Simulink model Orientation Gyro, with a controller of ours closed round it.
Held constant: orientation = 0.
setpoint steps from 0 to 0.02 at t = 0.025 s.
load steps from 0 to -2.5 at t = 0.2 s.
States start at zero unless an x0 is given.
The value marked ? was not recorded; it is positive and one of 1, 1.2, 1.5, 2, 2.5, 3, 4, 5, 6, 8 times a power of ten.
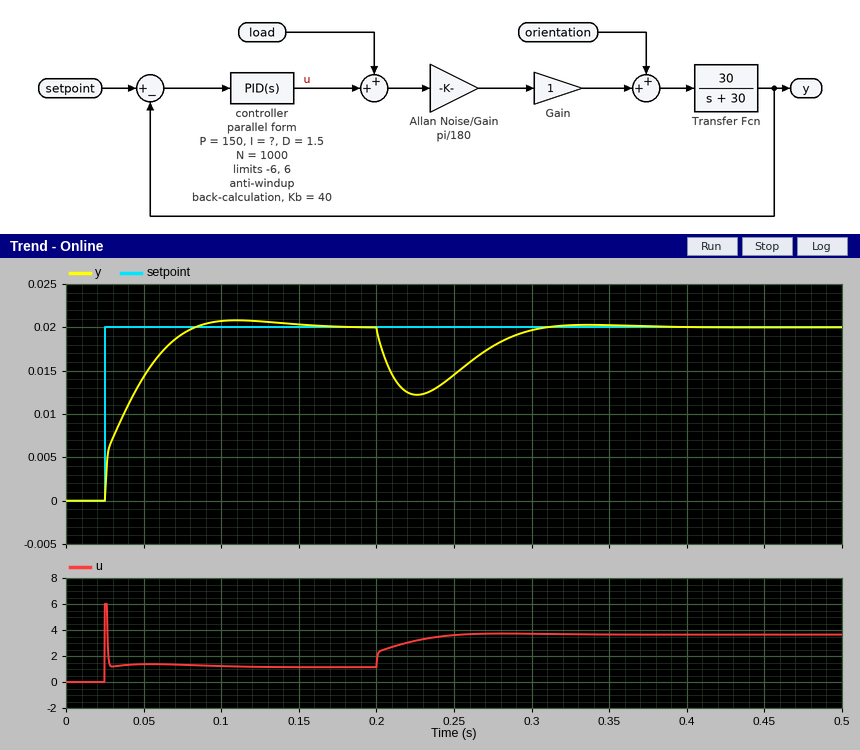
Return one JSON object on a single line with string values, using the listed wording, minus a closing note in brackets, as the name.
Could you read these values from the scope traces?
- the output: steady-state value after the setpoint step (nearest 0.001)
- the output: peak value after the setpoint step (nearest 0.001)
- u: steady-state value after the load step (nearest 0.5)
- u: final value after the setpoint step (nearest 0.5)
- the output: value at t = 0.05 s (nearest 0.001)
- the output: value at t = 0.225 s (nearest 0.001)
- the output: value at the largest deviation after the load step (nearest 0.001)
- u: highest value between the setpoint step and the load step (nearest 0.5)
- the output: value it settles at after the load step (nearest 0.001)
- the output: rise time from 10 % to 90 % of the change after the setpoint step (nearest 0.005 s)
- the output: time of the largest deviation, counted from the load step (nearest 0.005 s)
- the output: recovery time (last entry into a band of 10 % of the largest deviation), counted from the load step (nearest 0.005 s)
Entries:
{"the output: steady-state value after the setpoint step": "0.020", "the output: peak value after the setpoint step": "0.021", "u: steady-state value after the load step": "3.5", "u: final value after the setpoint step": "1.0", "the output: value at t = 0.05 s": "0.014", "the output: value at t = 0.225 s": "0.012", "the output: value at the largest deviation after the load step": "0.012", "u: highest value between the setpoint step and the load step": "6.0", "the output: value it settles at after the load step": "0.020", "the output: rise time from 10 % to 90 % of the change after the setpoint step": "0.040 s", "the output: time of the largest deviation, counted from the load step": "0.025 s", "the output: recovery time (last entry into a band of 10 % of the largest deviation), counted from the load step": "0.090 s"}
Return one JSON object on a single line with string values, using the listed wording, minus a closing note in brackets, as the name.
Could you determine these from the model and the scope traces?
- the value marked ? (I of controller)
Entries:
{"the value marked ?": "6000"}
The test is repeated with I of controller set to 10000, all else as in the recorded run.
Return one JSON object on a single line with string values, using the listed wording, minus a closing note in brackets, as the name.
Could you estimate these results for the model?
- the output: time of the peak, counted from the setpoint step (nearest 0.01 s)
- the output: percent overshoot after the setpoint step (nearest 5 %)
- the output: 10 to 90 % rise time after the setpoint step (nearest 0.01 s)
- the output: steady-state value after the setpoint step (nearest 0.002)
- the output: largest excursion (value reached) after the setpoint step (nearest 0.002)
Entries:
{"the output: time of the peak, counted from the setpoint step": "0.06 s", "the output: percent overshoot after the setpoint step": "10 %", "the output: 10 to 90 % rise time after the setpoint step": "0.03 s", "the output: steady-state value after the setpoint step": "0.020", "the output: largest excursion (value reached) after the setpoint step": "0.022"}
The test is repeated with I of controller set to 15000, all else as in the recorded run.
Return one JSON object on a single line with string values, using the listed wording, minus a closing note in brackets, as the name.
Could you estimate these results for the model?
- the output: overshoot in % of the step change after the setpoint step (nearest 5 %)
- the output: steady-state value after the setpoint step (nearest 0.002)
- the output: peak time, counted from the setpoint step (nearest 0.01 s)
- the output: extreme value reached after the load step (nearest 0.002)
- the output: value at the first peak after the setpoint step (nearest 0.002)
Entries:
{"the output: overshoot in % of the step change after the setpoint step": "15 %", "the output: steady-state value after the setpoint step": "0.020", "the output: peak time, counted from the setpoint step": "0.05 s", "the output: extreme value reached after the load step": "0.014", "the output: value at the first peak after the setpoint step": "0.024"}
